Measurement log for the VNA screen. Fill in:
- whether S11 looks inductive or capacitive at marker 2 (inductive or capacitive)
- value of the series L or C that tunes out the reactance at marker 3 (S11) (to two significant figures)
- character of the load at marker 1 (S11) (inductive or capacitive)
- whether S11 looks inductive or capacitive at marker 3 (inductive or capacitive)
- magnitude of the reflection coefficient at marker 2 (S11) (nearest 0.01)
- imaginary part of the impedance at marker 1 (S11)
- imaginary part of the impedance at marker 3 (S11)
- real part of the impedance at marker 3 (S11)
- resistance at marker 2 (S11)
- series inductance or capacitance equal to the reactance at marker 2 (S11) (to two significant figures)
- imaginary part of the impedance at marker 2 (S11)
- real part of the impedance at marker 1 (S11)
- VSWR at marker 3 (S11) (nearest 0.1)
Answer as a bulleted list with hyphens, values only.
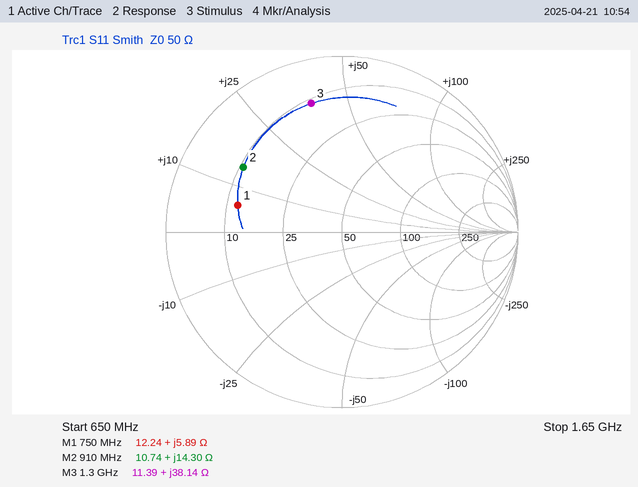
- inductive
- 3.2 pF
- inductive
- inductive
- 0.67
- +5.89 Ω
- +38.14 Ω
- 11.39 Ω
- 10.74 Ω
- 2.5 nH
- +14.30 Ω
- 12.24 Ω
- 7.0
